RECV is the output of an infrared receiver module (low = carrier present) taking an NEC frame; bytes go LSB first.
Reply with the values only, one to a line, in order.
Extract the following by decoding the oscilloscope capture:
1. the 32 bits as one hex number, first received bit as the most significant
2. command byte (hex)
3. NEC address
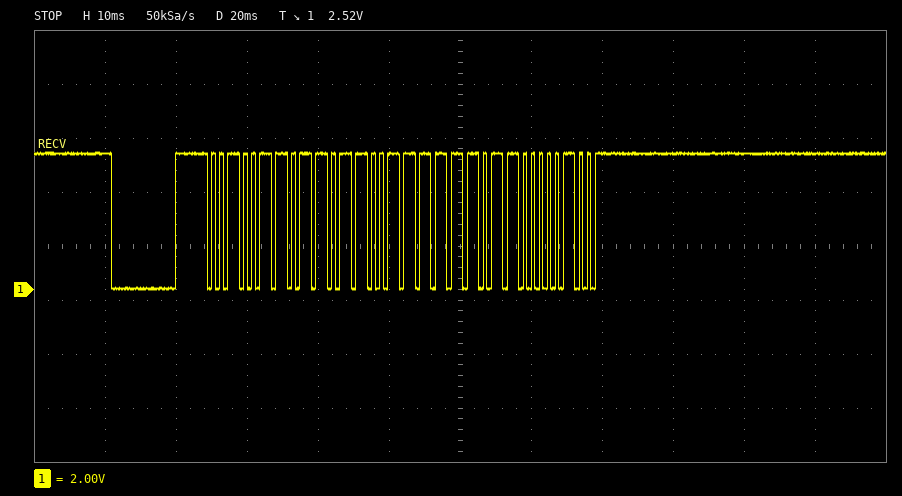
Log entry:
0x26D9FB04
0xDF
0x64
